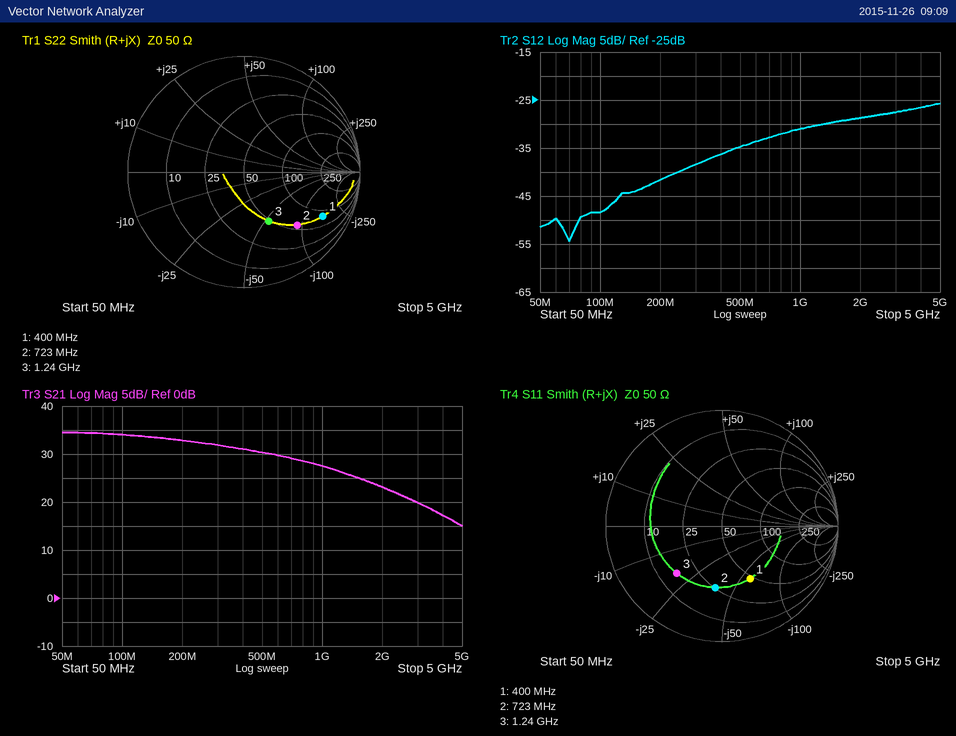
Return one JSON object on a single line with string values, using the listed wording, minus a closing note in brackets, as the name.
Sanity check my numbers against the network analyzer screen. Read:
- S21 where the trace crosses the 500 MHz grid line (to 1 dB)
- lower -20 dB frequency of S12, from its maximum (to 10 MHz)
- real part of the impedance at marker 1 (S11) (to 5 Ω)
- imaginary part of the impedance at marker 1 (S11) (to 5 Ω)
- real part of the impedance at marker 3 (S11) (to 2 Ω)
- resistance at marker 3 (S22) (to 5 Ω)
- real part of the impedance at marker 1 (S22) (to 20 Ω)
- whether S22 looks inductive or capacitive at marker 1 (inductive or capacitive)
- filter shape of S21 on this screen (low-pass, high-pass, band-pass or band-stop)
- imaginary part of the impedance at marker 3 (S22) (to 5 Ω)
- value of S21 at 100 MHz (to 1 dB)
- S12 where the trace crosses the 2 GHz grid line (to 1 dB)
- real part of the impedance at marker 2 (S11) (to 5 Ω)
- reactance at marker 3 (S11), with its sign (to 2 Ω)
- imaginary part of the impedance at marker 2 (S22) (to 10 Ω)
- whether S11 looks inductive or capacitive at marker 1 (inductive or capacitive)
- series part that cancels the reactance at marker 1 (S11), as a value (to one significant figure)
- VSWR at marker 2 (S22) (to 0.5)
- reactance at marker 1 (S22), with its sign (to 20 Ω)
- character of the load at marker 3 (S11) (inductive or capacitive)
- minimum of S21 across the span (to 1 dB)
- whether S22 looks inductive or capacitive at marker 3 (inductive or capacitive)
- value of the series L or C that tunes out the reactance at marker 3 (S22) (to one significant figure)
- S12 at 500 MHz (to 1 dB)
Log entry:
{"S21 where the trace crosses the 500 MHz grid line": "30 dB", "lower -20 dB frequency of S12, from its maximum": "120 MHz", "real part of the impedance at marker 1 (S11)": "45 Ω", "imaginary part of the impedance at marker 1 (S11)": "-60 Ω", "real part of the impedance at marker 3 (S11)": "16 Ω", "resistance at marker 3 (S22)": "50 Ω", "real part of the impedance at marker 1 (S22)": "80 Ω", "whether S22 looks inductive or capacitive at marker 1": "capacitive", "filter shape of S21 on this screen": "low-pass", "imaginary part of the impedance at marker 3 (S22)": "-55 Ω", "value of S21 at 100 MHz": "34 dB", "S12 where the trace crosses the 2 GHz grid line": "-29 dB", "real part of the impedance at marker 2 (S11)": "25 Ω", "reactance at marker 3 (S11), with its sign": "-20 Ω", "imaginary part of the impedance at marker 2 (S22)": "-90 Ω", "whether S11 looks inductive or capacitive at marker 1": "capacitive", "series part that cancels the reactance at marker 1 (S11), as a value": "20 nH", "VSWR at marker 2 (S22)": "4.5", "reactance at marker 1 (S22), with its sign": "-160 Ω", "character of the load at marker 3 (S11)": "capacitive", "minimum of S21 across the span": "15 dB", "whether S22 looks inductive or capacitive at marker 3": "capacitive", "value of the series L or C that tunes out the reactance at marker 3 (S22)": "7 nH", "S12 at 500 MHz": "-35 dB"}
